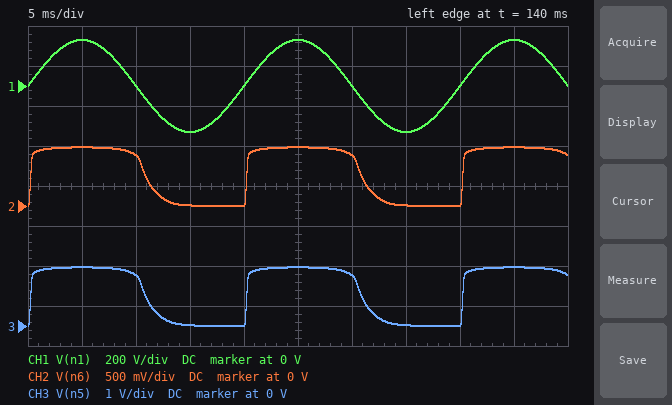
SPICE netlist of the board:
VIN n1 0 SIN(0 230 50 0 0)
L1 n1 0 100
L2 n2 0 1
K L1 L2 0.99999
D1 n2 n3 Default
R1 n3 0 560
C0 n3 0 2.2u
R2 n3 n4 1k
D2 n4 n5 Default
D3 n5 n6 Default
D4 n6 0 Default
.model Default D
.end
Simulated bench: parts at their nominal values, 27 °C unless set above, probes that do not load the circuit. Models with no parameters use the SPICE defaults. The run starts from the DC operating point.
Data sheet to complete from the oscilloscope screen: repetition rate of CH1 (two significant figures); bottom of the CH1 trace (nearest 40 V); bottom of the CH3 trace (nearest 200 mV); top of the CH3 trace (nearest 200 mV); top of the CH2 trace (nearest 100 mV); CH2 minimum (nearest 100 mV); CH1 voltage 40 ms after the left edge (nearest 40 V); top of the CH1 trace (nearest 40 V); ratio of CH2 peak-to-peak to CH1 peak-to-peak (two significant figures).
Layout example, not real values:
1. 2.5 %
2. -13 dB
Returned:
1. 50 Hz
2. -240 V
3. 0 V
4. 1.4 V
5. 700 mV
6. 0 V
7. 0 V
8. 240 V
9. 0.0016
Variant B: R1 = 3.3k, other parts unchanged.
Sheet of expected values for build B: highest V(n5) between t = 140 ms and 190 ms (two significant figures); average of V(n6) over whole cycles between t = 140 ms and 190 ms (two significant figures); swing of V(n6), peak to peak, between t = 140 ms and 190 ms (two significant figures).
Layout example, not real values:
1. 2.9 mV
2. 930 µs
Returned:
1. 1.5 V
2. 600 mV
3. 480 mV
